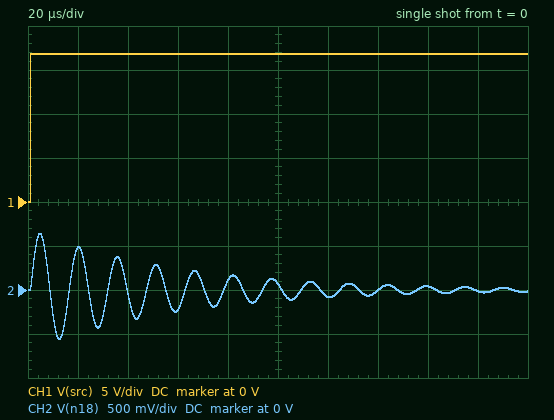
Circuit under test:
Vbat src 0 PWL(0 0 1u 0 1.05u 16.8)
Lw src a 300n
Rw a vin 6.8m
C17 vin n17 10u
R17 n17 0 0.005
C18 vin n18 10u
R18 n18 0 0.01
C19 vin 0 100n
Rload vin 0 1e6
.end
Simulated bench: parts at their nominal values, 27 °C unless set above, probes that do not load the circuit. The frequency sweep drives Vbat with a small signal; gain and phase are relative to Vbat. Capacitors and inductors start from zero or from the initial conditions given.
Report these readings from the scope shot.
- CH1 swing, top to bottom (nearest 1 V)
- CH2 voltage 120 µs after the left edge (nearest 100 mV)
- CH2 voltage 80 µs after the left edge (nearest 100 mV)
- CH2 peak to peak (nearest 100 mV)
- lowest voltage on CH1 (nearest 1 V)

17 V
-100 mV
100 mV
1.2 V
0 V
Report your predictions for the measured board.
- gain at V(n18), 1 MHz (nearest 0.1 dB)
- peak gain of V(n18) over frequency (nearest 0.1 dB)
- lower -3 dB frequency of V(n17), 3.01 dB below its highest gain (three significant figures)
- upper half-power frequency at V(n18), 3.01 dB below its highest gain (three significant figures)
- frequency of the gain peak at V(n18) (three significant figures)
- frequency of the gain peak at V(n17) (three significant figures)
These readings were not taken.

-52.0 dB
-6.5 dB
62.1 kHz
67.7 kHz
64.8 kHz
64.8 kHz
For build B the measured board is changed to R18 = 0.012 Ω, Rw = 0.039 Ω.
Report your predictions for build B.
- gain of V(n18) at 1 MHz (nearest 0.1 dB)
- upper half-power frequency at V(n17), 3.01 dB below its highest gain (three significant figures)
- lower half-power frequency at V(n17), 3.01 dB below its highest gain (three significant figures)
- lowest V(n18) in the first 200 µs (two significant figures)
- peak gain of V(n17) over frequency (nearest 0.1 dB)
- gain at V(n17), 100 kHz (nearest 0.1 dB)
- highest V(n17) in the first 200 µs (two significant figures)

-50.6 dB
77.3 kHz
54.4 kHz
-360 mV
-24.8 dB
-33.5 dB
270 mV
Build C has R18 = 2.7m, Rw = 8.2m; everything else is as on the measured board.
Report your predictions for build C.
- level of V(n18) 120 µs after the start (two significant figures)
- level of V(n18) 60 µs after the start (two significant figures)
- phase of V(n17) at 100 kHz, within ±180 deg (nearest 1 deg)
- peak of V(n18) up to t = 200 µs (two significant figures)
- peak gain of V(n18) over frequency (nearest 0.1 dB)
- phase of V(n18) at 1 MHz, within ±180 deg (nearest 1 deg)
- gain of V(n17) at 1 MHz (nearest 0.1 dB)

-24 mV
-62 mV
-85 deg
170 mV
-17.5 dB
-86 deg
-57.7 dB
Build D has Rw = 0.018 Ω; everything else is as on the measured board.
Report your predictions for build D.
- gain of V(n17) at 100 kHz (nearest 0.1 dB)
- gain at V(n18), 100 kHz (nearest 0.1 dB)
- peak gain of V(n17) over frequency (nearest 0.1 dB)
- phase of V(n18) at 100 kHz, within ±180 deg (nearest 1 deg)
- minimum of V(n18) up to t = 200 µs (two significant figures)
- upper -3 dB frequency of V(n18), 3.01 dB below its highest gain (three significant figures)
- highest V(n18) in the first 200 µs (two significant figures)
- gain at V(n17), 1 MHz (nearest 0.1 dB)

-33.0 dB
-27.0 dB
-18.8 dB
-80 deg
-450 mV
70.8 kHz
600 mV
-57.0 dB
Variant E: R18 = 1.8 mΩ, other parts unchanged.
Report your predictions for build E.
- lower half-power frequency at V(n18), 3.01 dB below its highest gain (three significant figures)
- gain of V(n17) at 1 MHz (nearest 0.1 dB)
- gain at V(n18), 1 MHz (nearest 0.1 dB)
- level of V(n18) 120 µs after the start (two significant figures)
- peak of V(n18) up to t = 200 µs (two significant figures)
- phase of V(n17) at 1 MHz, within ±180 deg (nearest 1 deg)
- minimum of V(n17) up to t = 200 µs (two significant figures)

62.6 kHz
-57.7 dB
-66.2 dB
-22 mV
120 mV
-95 deg
-290 mV
